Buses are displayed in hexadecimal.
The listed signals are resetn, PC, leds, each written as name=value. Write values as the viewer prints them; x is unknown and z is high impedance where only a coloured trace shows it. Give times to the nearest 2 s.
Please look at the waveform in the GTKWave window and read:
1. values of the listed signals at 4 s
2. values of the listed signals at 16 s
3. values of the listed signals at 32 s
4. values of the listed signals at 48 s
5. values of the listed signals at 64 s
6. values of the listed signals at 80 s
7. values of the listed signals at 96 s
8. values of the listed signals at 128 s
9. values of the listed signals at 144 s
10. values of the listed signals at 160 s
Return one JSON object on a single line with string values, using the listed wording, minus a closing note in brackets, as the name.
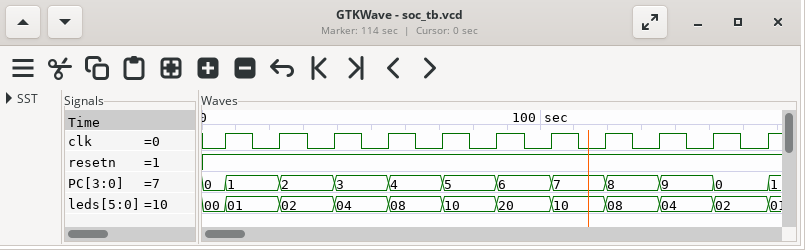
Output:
{"values of the listed signals at 4 s": "resetn=1, PC=0, leds=00", "values of the listed signals at 16 s": "resetn=1, PC=1, leds=01", "values of the listed signals at 32 s": "resetn=1, PC=2, leds=02", "values of the listed signals at 48 s": "resetn=1, PC=3, leds=04", "values of the listed signals at 64 s": "resetn=1, PC=4, leds=08", "values of the listed signals at 80 s": "resetn=1, PC=5, leds=10", "values of the listed signals at 96 s": "resetn=1, PC=6, leds=20", "values of the listed signals at 128 s": "resetn=1, PC=8, leds=08", "values of the listed signals at 144 s": "resetn=1, PC=9, leds=04", "values of the listed signals at 160 s": "resetn=1, PC=0, leds=02"}
